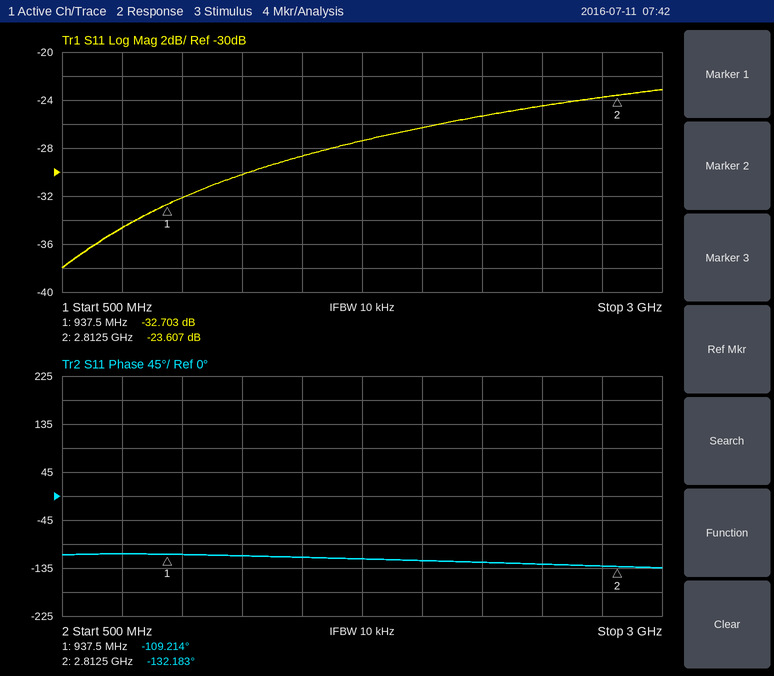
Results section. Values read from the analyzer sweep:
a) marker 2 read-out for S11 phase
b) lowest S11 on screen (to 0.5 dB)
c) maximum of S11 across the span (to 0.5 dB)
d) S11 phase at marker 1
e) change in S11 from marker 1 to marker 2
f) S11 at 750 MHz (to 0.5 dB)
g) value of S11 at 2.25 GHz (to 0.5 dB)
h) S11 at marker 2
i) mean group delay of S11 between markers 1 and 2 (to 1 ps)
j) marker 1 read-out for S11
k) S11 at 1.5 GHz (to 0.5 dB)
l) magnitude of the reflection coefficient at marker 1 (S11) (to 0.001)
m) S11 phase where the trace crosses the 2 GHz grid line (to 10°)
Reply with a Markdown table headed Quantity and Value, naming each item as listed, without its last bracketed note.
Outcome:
| Quantity | Value |
|---|---|
| marker 2 read-out for S11 phase | -132.183° |
| lowest S11 on screen | -38.0 dB |
| maximum of S11 across the span | -23.0 dB |
| S11 phase at marker 1 | -109.214° |
| change in S11 from marker 1 to marker 2 | 9.096 dB |
| S11 at 750 MHz | -34.5 dB |
| value of S11 at 2.25 GHz | -25.5 dB |
| S11 at marker 2 | -23.607 dB |
| mean group delay of S11 between markers 1 and 2 | 34 ps |
| marker 1 read-out for S11 | -32.703 dB |
| S11 at 1.5 GHz | -28.5 dB |
| magnitude of the reflection coefficient at marker 1 (S11) | 0.023 |
| S11 phase where the trace crosses the 2 GHz grid line | -120° |
